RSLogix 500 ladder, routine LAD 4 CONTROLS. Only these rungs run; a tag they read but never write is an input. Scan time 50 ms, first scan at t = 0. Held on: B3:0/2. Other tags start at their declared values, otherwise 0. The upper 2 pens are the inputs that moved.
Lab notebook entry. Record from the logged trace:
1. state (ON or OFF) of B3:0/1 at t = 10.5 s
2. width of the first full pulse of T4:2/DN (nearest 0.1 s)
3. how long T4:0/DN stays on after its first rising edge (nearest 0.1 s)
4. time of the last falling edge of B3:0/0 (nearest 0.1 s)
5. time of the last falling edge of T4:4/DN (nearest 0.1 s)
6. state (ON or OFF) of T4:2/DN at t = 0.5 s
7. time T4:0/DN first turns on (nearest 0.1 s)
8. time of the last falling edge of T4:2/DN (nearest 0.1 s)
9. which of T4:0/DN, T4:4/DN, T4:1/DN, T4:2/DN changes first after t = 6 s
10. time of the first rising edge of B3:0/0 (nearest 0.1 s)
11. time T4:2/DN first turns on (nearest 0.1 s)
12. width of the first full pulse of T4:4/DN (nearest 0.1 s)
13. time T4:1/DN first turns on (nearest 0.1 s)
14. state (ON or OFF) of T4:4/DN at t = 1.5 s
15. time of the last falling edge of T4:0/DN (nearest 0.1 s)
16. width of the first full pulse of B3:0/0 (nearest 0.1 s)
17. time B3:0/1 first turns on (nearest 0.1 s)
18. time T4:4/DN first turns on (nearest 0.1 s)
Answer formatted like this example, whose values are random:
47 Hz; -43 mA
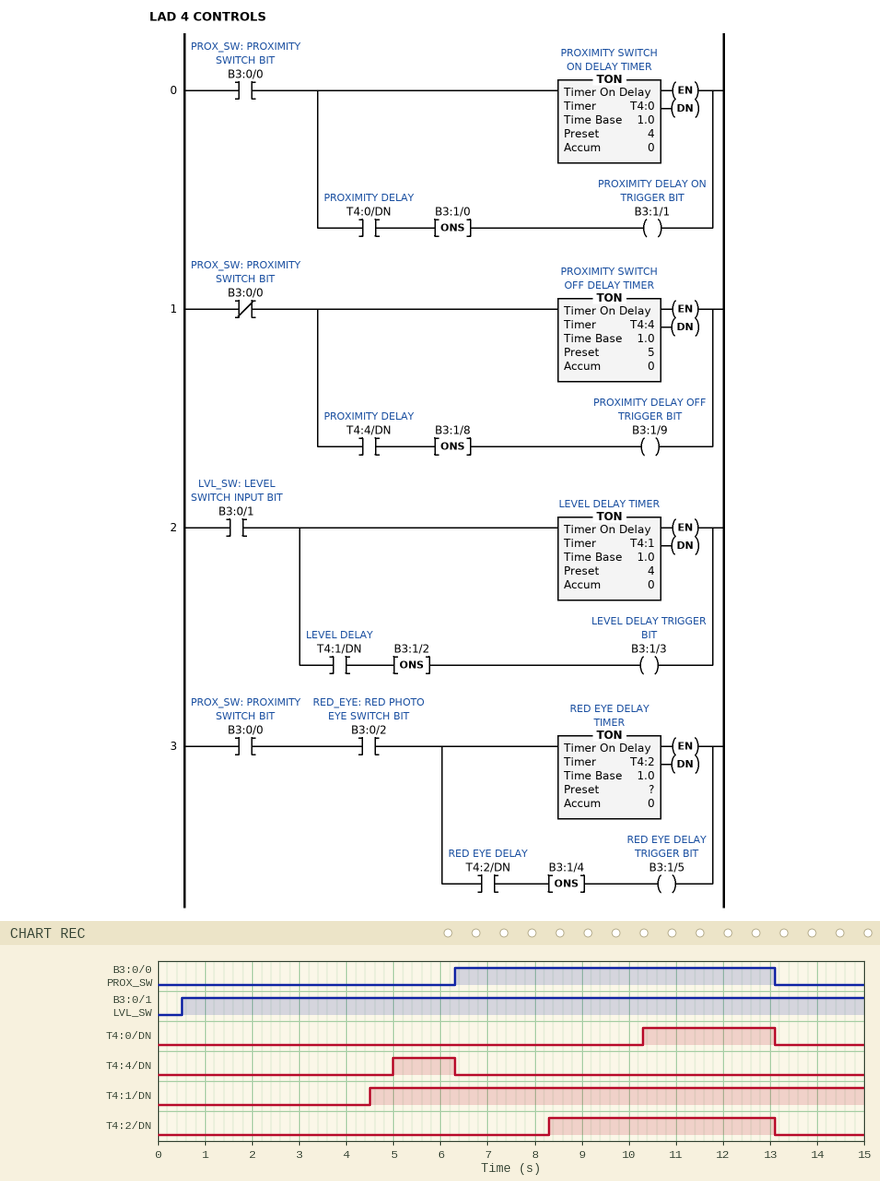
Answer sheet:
ON; 4.8 s; 2.8 s; 13.1 s; 6.3 s; OFF; 10.3 s; 13.1 s; T4:4/DN; 6.3 s; 8.3 s; 1.3 s; 4.5 s; OFF; 13.1 s; 6.8 s; 0.5 s; 5.0 s
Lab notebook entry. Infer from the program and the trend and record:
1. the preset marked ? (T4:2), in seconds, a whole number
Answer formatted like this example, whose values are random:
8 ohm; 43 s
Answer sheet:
2 s
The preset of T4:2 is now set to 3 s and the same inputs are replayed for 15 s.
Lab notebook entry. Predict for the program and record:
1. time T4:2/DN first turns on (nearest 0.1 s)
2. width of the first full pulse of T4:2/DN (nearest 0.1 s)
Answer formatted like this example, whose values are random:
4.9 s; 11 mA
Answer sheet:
9.3 s; 3.8 s
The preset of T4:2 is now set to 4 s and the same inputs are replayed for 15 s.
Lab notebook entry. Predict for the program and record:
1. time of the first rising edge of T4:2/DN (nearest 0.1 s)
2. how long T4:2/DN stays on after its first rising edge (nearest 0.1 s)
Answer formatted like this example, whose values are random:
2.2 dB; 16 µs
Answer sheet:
10.3 s; 2.8 s
